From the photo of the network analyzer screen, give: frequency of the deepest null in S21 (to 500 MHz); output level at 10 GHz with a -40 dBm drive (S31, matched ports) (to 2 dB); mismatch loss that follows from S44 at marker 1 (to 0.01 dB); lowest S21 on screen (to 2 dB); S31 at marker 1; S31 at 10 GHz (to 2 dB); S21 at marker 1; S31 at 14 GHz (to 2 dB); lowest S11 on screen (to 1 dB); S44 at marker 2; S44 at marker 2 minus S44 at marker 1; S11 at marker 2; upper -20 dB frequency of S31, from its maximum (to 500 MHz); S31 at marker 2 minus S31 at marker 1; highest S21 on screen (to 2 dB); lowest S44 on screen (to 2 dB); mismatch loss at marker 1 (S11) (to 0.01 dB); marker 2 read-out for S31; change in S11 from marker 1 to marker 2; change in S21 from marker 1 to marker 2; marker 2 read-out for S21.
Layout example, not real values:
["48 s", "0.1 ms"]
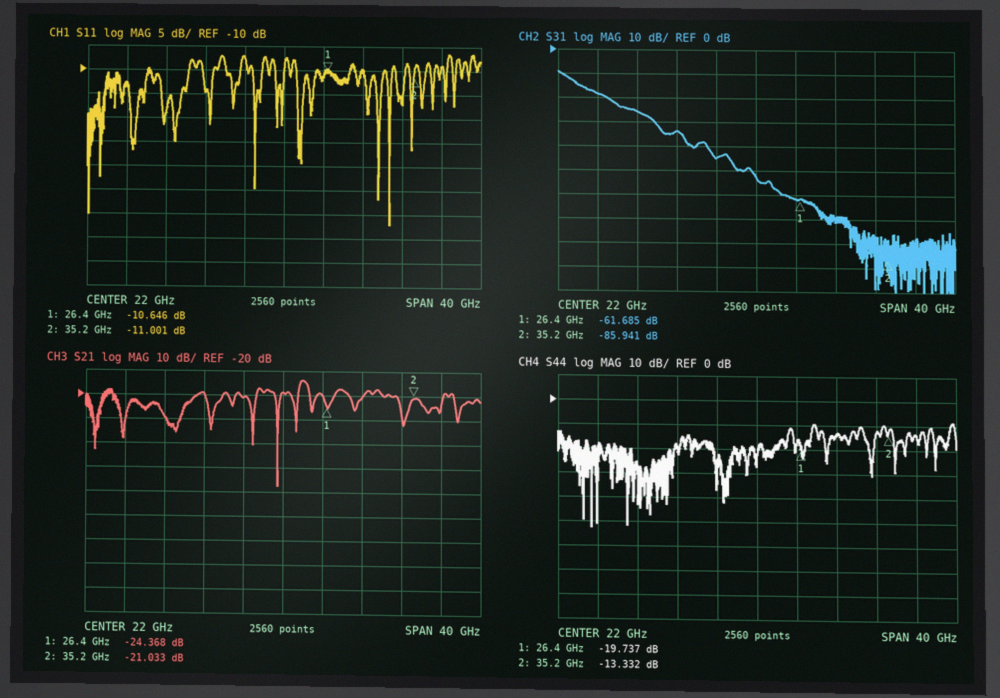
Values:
["21.5 GHz", "-66 dBm", "0.05 dB", "-58 dB", "-61.685 dB", "-26 dB", "-24.368 dB", "-34 dB", "-42 dB", "-13.332 dB", "6.405 dB", "-11.001 dB", "11.5 GHz", "-24.256 dB", "-14 dB", "-52 dB", "0.39 dB", "-85.941 dB", "-0.355 dB", "3.335 dB", "-21.033 dB"]
